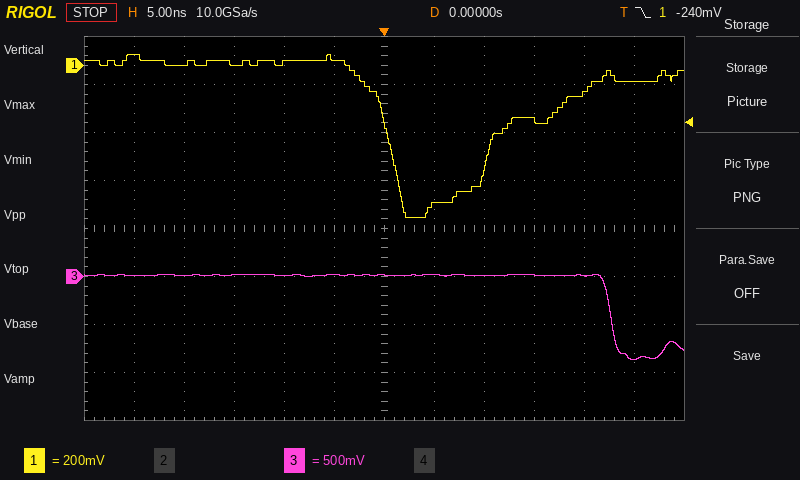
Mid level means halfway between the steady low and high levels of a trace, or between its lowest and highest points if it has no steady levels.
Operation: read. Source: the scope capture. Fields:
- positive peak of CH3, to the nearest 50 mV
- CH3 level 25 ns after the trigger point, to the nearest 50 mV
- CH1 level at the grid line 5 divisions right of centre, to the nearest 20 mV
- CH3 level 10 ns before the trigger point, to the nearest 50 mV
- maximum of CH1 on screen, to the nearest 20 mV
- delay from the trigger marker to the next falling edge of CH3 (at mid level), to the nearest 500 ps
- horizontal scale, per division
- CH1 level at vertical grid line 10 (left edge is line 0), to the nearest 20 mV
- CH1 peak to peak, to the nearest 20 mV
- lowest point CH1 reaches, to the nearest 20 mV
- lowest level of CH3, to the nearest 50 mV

0 mV
-850 mV
-60 mV
0 mV
40 mV
22.5 ns
5 ns
-120 mV
680 mV
-640 mV
-850 mV
